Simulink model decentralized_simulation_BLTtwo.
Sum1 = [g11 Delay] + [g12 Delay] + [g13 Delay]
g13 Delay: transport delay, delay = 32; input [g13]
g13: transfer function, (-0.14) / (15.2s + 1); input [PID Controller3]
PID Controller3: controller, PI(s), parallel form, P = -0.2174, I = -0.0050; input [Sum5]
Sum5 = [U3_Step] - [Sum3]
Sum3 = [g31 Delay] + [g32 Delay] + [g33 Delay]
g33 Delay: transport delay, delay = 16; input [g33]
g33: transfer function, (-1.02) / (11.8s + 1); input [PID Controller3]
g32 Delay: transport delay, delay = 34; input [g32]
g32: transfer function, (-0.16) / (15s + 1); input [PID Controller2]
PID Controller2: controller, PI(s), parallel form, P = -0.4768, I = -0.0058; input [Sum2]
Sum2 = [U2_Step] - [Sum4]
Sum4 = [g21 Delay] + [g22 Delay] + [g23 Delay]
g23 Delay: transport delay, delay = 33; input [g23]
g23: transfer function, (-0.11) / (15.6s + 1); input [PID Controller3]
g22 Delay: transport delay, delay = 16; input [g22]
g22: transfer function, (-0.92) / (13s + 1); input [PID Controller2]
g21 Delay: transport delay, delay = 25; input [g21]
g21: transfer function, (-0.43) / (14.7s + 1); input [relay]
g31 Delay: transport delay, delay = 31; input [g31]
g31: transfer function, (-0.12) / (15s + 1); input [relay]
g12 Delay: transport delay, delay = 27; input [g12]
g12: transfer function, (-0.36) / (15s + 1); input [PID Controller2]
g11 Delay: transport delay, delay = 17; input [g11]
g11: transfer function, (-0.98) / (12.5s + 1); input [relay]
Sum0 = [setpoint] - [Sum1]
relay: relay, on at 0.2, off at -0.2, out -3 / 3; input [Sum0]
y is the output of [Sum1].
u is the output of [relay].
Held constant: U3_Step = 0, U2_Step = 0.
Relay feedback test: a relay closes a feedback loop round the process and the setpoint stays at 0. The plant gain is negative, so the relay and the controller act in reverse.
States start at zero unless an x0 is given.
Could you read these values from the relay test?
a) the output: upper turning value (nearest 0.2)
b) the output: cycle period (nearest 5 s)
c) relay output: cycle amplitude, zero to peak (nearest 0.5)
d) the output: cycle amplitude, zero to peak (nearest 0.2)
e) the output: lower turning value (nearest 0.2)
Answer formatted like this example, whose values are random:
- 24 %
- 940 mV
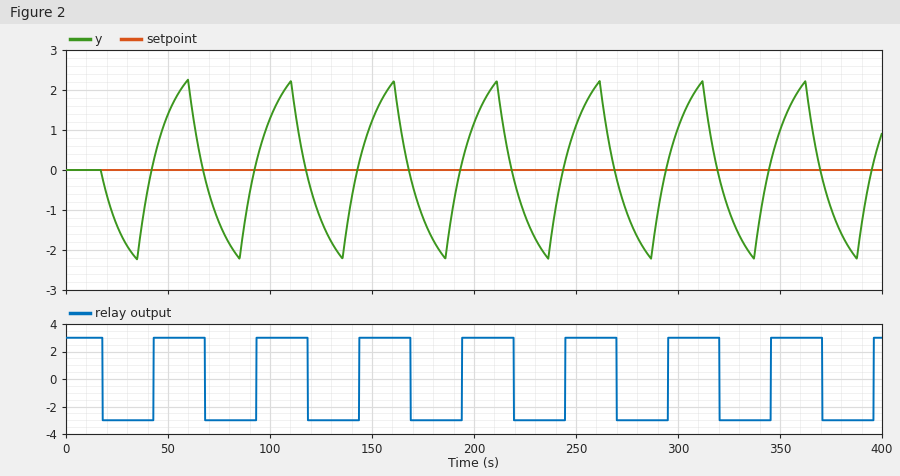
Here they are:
- 2.2
- 50 s
- 3.0
- 2.2
- -2.2
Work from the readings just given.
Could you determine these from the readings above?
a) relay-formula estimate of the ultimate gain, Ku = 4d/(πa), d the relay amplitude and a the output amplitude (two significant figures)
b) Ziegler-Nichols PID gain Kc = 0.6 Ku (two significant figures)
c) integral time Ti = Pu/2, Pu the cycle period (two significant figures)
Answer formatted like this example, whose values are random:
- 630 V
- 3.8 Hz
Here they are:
- 1.7
- 1.0
- 25 s
